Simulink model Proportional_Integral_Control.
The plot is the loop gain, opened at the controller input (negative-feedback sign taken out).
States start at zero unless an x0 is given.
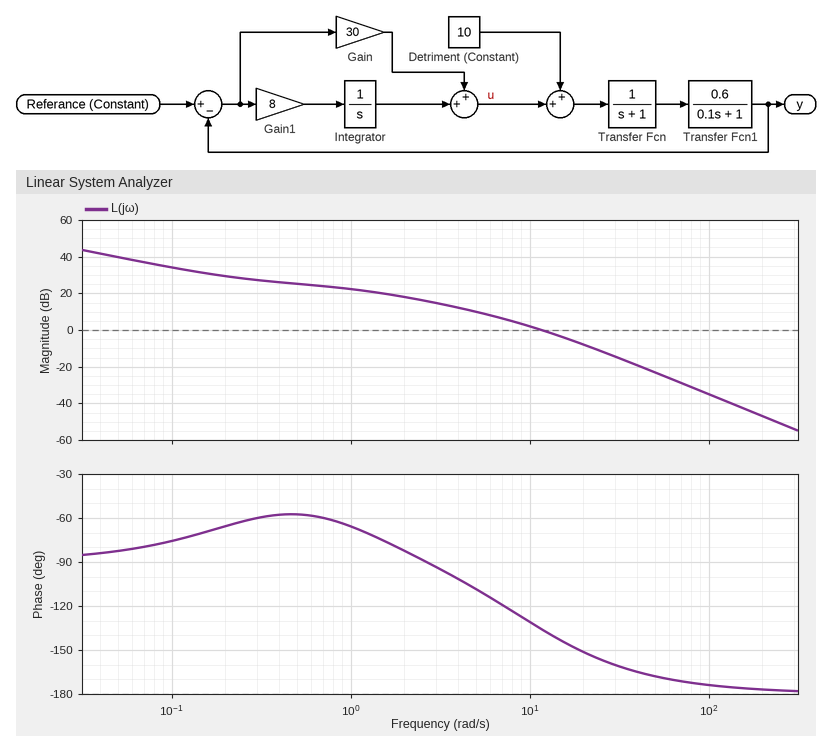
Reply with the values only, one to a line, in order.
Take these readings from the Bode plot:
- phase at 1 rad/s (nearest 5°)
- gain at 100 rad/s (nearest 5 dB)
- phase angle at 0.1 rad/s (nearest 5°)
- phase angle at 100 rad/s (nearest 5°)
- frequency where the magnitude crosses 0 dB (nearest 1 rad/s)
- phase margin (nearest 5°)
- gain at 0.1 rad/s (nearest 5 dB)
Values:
-65°
-35 dB
-75°
-175°
12 rad/s
45°
35 dB
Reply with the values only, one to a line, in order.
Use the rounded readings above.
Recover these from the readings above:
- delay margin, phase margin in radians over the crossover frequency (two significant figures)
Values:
0.065 s
